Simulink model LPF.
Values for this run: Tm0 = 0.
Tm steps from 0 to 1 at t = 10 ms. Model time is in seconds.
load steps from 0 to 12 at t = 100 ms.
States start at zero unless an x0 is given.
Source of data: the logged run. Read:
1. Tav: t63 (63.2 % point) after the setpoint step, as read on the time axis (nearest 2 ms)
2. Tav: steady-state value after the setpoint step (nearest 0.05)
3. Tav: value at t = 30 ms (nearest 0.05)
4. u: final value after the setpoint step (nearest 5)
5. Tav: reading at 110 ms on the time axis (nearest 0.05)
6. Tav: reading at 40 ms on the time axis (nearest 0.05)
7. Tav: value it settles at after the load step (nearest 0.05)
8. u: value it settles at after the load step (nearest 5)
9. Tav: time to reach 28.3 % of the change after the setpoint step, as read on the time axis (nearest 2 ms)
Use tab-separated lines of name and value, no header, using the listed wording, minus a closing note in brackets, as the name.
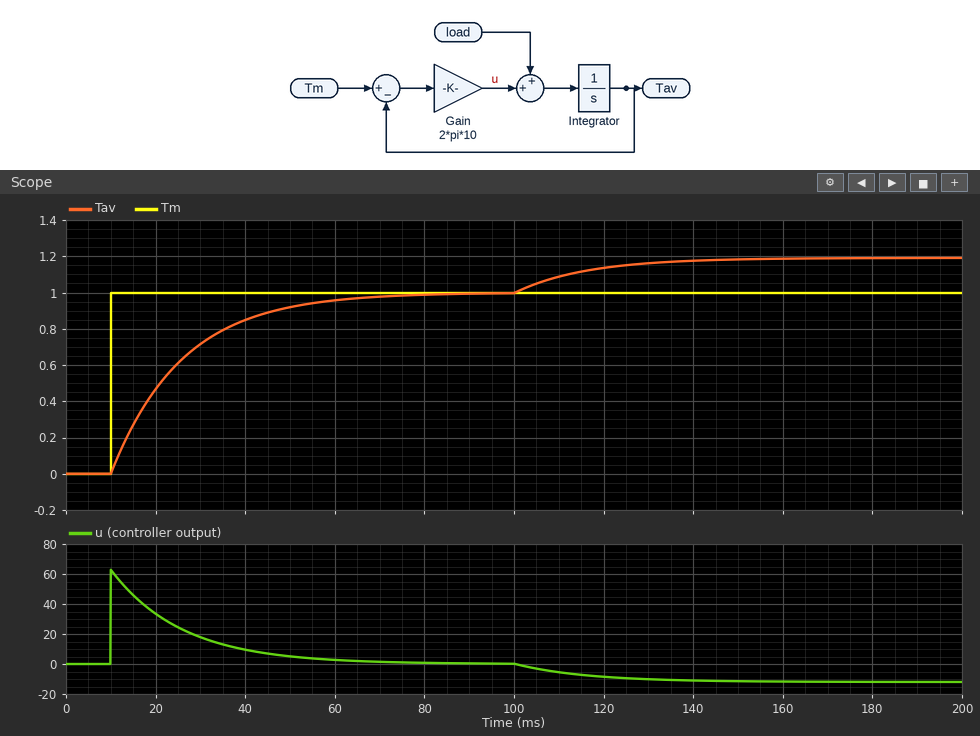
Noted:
Tav: t63 (63.2 % point) after the setpoint step, as read on the time axis	26 ms
Tav: steady-state value after the setpoint step	1.00
Tav: value at t = 30 ms	0.70
u: final value after the setpoint step	0
Tav: reading at 110 ms on the time axis	1.10
Tav: reading at 40 ms on the time axis	0.85
Tav: value it settles at after the load step	1.20
u: value it settles at after the load step	-10
Tav: time to reach 28.3 % of the change after the setpoint step, as read on the time axis	16 ms
